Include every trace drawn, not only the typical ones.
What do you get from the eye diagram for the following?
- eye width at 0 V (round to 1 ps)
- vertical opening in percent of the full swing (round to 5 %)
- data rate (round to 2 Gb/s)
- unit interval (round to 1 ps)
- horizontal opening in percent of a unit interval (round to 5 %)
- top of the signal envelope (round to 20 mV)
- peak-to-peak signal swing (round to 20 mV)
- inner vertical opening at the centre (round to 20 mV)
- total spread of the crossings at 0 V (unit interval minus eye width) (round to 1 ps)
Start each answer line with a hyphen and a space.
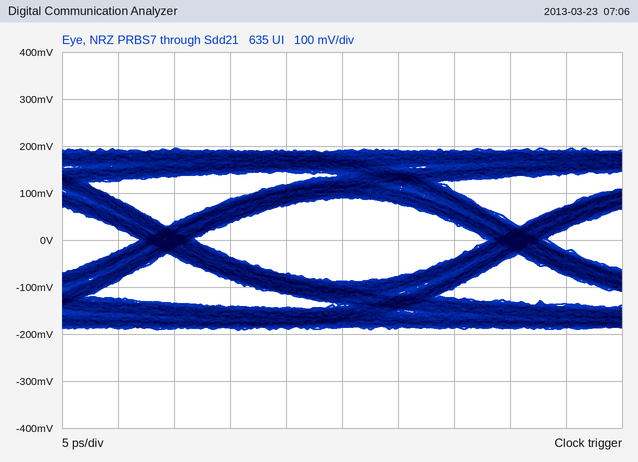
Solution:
- 26 ps
- 45 %
- 32 Gb/s
- 31 ps
- 85 %
- 200 mV
- 380 mV
- 180 mV
- 5 ps
